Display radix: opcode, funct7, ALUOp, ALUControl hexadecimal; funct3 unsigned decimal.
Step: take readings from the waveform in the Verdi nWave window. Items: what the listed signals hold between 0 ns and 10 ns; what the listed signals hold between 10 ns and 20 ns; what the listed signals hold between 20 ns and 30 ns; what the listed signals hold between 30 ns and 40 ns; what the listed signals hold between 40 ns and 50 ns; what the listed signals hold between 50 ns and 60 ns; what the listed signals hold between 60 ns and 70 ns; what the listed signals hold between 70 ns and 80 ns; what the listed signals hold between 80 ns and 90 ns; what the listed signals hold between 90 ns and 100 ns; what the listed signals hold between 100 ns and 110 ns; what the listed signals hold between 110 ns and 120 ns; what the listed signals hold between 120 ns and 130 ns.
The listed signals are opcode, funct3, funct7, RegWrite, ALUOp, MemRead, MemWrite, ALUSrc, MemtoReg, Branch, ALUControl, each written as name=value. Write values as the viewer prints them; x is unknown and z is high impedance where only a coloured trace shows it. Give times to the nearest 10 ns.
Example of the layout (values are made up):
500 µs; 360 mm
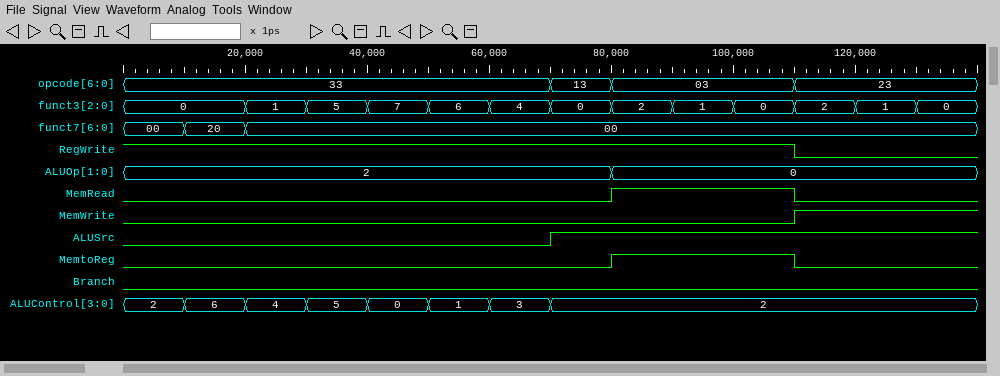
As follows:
opcode=33, funct3=0, funct7=00, RegWrite=1, ALUOp=2, MemRead=0, MemWrite=0, ALUSrc=0, MemtoReg=0, Branch=0, ALUControl=2; opcode=33, funct3=0, funct7=20, RegWrite=1, ALUOp=2, MemRead=0, MemWrite=0, ALUSrc=0, MemtoReg=0, Branch=0, ALUControl=6; opcode=33, funct3=1, funct7=00, RegWrite=1, ALUOp=2, MemRead=0, MemWrite=0, ALUSrc=0, MemtoReg=0, Branch=0, ALUControl=4; opcode=33, funct3=5, funct7=00, RegWrite=1, ALUOp=2, MemRead=0, MemWrite=0, ALUSrc=0, MemtoReg=0, Branch=0, ALUControl=5; opcode=33, funct3=7, funct7=00, RegWrite=1, ALUOp=2, MemRead=0, MemWrite=0, ALUSrc=0, MemtoReg=0, Branch=0, ALUControl=0; opcode=33, funct3=6, funct7=00, RegWrite=1, ALUOp=2, MemRead=0, MemWrite=0, ALUSrc=0, MemtoReg=0, Branch=0, ALUControl=1; opcode=33, funct3=4, funct7=00, RegWrite=1, ALUOp=2, MemRead=0, MemWrite=0, ALUSrc=0, MemtoReg=0, Branch=0, ALUControl=3; opcode=13, funct3=0, funct7=00, RegWrite=1, ALUOp=2, MemRead=0, MemWrite=0, ALUSrc=1, MemtoReg=0, Branch=0, ALUControl=2; opcode=03, funct3=2, funct7=00, RegWrite=1, ALUOp=0, MemRead=1, MemWrite=0, ALUSrc=1, MemtoReg=1, Branch=0, ALUControl=2; opcode=03, funct3=1, funct7=00, RegWrite=1, ALUOp=0, MemRead=1, MemWrite=0, ALUSrc=1, MemtoReg=1, Branch=0, ALUControl=2; opcode=03, funct3=0, funct7=00, RegWrite=1, ALUOp=0, MemRead=1, MemWrite=0, ALUSrc=1, MemtoReg=1, Branch=0, ALUControl=2; opcode=23, funct3=2, funct7=00, RegWrite=0, ALUOp=0, MemRead=0, MemWrite=1, ALUSrc=1, MemtoReg=0, Branch=0, ALUControl=2; opcode=23, funct3=1, funct7=00, RegWrite=0, ALUOp=0, MemRead=0, MemWrite=1, ALUSrc=1, MemtoReg=0, Branch=0, ALUControl=2
